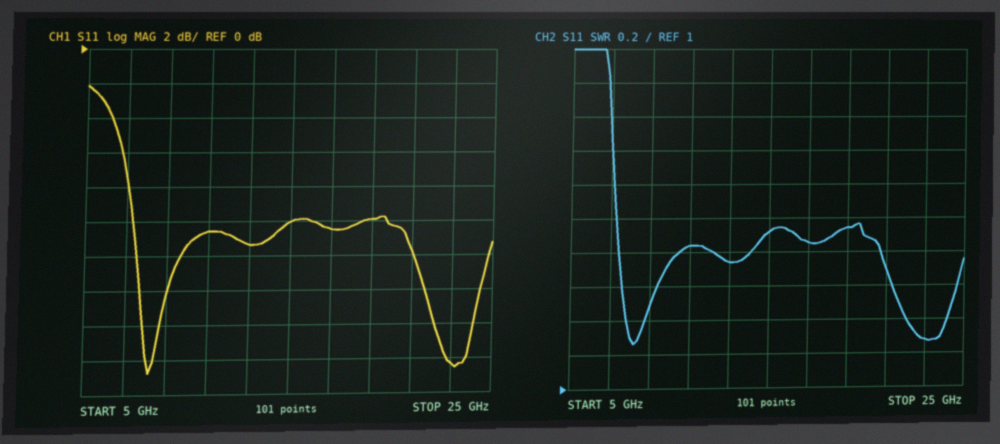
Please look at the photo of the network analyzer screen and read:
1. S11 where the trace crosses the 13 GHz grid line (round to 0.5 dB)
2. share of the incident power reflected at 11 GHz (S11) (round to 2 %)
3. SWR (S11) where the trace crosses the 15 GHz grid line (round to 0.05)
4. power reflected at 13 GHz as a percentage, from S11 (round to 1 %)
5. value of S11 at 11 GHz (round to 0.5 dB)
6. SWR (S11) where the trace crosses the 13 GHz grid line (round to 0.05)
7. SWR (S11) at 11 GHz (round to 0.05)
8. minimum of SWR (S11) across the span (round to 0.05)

-11.5 dB
8 %
1.90
7 %
-10.5 dB
1.75
1.85
1.25
